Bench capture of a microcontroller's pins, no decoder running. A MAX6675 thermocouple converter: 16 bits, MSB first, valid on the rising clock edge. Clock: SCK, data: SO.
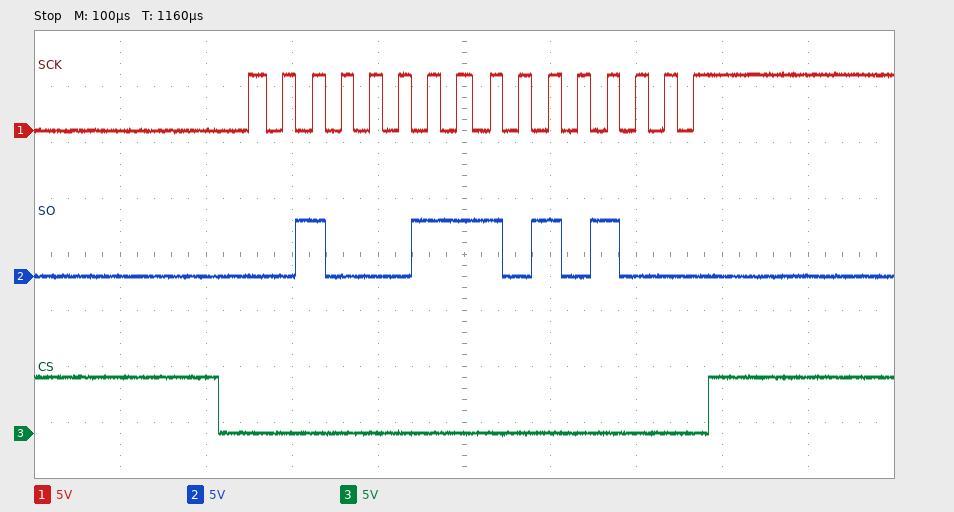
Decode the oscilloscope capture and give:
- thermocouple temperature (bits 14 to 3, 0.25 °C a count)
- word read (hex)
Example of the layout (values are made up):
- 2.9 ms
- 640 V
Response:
- 285.25 °C
- 0x23A8
